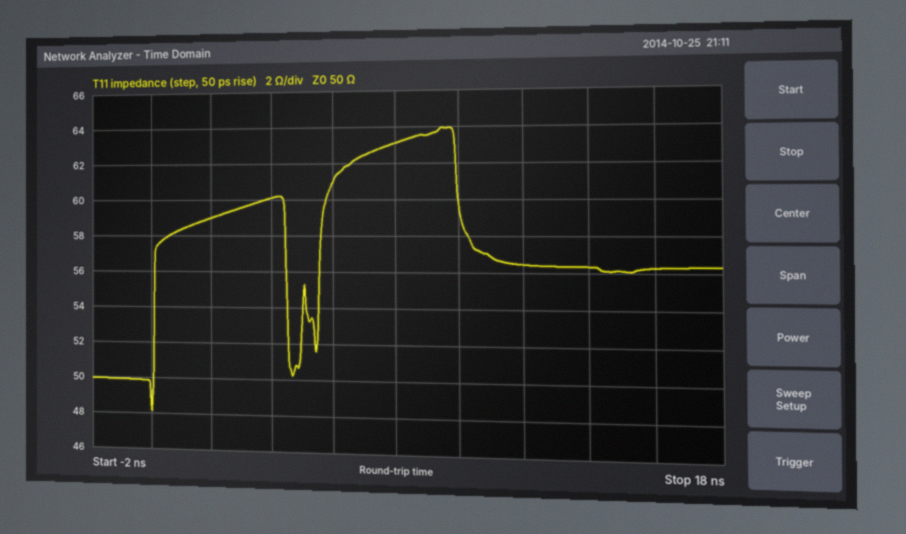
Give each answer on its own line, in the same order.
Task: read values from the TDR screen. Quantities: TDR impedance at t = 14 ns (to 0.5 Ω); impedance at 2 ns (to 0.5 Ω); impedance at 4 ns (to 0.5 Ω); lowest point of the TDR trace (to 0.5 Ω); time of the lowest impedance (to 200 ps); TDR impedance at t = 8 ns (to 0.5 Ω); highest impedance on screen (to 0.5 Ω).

56.5 Ω
59.0 Ω
60.0 Ω
48.0 Ω
0.0 ns
63.0 Ω
64.0 Ω
